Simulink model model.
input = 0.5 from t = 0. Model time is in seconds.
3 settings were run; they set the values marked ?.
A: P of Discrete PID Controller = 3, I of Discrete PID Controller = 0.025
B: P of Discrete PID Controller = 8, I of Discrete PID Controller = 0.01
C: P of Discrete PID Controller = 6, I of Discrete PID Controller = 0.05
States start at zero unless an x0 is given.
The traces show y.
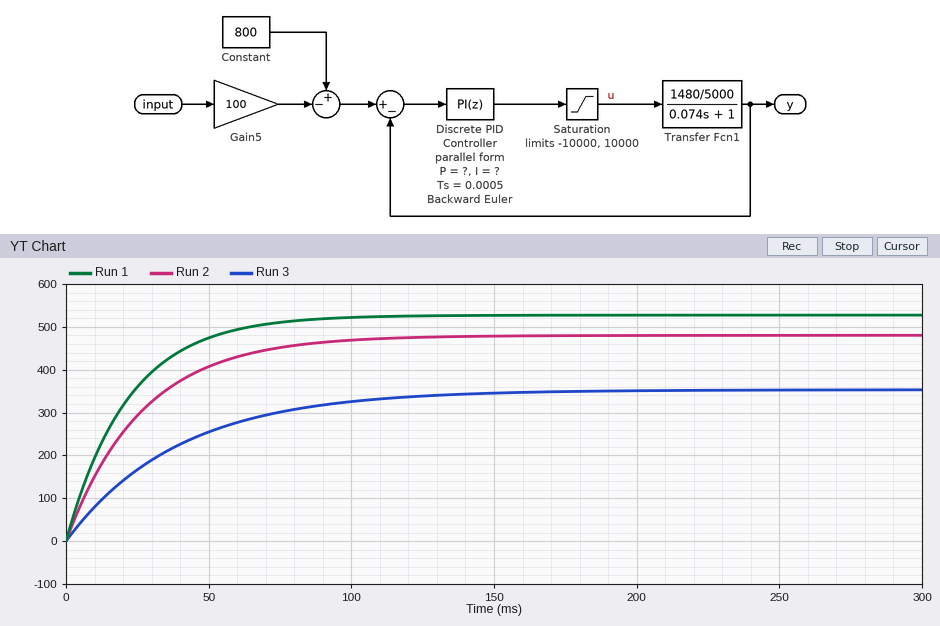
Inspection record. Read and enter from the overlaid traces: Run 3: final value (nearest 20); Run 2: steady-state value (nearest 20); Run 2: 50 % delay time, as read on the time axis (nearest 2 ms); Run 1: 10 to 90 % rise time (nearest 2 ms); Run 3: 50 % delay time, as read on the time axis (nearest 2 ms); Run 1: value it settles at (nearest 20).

360
480
18 ms
48 ms
28 ms
520
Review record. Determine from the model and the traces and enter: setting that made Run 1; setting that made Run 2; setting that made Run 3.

B
C
A
